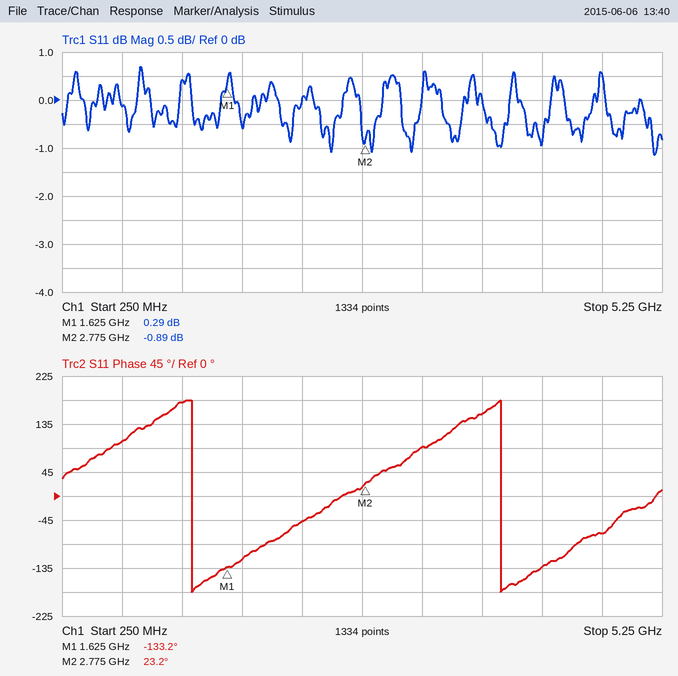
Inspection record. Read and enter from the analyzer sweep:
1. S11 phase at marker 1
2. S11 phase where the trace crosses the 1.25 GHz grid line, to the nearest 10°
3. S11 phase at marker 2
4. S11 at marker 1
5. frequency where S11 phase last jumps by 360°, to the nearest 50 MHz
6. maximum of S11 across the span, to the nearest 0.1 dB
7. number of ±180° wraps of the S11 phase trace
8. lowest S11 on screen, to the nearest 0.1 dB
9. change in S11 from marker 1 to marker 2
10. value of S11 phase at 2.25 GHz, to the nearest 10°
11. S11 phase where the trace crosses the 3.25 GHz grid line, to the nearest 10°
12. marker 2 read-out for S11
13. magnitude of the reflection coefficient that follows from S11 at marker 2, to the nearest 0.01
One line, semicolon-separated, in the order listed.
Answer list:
-133.2°; 180°; 23.2°; 0.29 dB; 3.90 GHz; 0.7 dB; 2; -1.1 dB; -1.18 dB; -50°; 90°; -0.89 dB; 0.90
